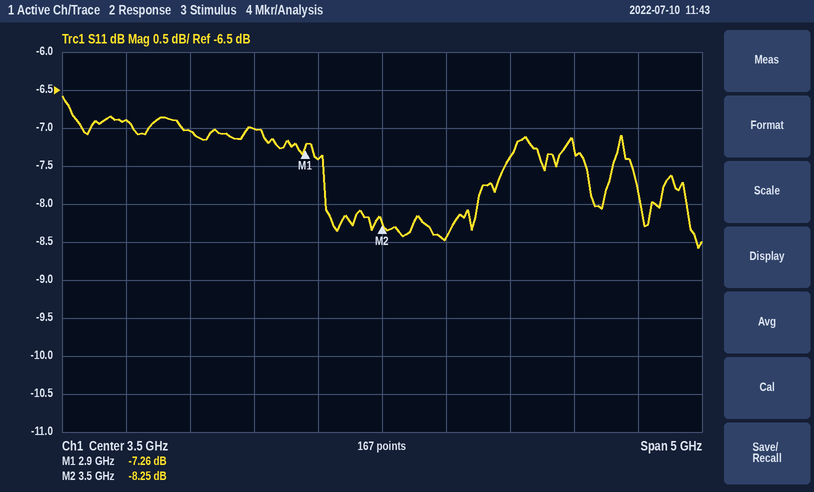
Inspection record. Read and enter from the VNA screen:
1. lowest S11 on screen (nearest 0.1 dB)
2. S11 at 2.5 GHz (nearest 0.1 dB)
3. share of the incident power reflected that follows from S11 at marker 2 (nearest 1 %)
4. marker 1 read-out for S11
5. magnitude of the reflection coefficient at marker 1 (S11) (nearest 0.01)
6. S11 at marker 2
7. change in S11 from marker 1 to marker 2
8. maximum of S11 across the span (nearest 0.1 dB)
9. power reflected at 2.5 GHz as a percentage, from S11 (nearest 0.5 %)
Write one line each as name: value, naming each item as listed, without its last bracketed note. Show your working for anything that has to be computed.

lowest S11 on screen: -8.6 dB
S11 at 2.5 GHz: -7.0 dB
share of the incident power reflected that follows from S11 at marker 2: 10^(-8.25/10) ≈ 15 %
marker 1 read-out for S11: -7.26 dB
magnitude of the reflection coefficient at marker 1 (S11): 10^(-7.26/20) ≈ 0.43
S11 at marker 2: -8.25 dB
change in S11 from marker 1 to marker 2: -8.25 − (-7.26) = -0.99 dB
maximum of S11 across the span: -6.6 dB
power reflected at 2.5 GHz as a percentage, from S11: 10^(-7/10) ≈ 20.0 %
